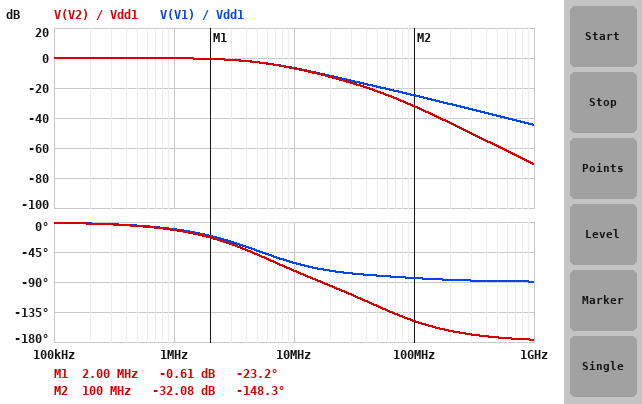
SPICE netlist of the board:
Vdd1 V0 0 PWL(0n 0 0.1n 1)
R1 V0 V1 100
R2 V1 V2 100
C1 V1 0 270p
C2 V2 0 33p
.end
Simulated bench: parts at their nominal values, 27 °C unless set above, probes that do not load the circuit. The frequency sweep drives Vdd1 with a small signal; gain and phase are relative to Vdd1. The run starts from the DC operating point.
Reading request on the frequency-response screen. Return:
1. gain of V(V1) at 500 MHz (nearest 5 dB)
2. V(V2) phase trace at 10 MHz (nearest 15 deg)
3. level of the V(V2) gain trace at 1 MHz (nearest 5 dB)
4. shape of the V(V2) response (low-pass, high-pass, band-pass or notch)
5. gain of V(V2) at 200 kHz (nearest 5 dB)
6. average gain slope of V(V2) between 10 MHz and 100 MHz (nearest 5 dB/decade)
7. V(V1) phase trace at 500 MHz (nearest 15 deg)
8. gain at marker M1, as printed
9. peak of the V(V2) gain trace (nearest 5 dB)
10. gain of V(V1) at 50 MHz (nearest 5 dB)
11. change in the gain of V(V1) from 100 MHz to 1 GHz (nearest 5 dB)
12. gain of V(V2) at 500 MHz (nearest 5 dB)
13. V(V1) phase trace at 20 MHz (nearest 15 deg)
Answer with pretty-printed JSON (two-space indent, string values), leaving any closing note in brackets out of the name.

{
  "gain of V(V1) at 500 MHz": "-40 dB",
  "V(V2) phase trace at 10 MHz": "-75 deg",
  "level of the V(V2) gain trace at 1 MHz": "0 dB",
  "shape of the V(V2) response": "low-pass",
  "gain of V(V2) at 200 kHz": "0 dB",
  "average gain slope of V(V2) between 10 MHz and 100 MHz": "-25 dB/decade",
  "V(V1) phase trace at 500 MHz": "-90 deg",
  "gain at marker M1, as printed": "-0.61 dB",
  "peak of the V(V2) gain trace": "0 dB",
  "gain of V(V1) at 50 MHz": "-20 dB",
  "change in the gain of V(V1) from 100 MHz to 1 GHz": "-20 dB",
  "gain of V(V2) at 500 MHz": "-60 dB",
  "V(V1) phase trace at 20 MHz": "-75 deg"
}
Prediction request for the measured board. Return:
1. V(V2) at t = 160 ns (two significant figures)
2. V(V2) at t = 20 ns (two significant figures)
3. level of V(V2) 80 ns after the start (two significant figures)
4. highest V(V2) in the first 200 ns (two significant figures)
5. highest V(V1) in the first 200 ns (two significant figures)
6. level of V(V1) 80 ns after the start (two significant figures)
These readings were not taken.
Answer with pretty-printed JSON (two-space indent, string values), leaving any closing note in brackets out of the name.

{
  "V(V2) at t = 160 ns": "990 mV",
  "V(V2) at t = 20 ns": "420 mV",
  "level of V(V2) 80 ns after the start": "920 mV",
  "highest V(V2) in the first 200 ns": "1.0 V",
  "highest V(V1) in the first 200 ns": "1.0 V",
  "level of V(V1) 80 ns after the start": "930 mV"
}
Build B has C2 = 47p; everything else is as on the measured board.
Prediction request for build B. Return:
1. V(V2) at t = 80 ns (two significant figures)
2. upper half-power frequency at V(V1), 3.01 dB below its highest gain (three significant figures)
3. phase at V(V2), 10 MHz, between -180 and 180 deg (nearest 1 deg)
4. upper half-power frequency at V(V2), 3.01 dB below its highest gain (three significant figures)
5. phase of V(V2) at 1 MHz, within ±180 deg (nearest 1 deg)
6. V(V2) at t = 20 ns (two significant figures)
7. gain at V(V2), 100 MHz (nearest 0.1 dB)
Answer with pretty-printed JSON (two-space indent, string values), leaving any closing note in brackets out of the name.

{
  "V(V2) at t = 80 ns": "900 mV",
  "upper half-power frequency at V(V1), 3.01 dB below its highest gain": "4.93 MHz",
  "phase at V(V2), 10 MHz, between -180 and 180 deg": "-78 deg",
  "upper half-power frequency at V(V2), 3.01 dB below its highest gain": "4.83 MHz",
  "phase of V(V2) at 1 MHz, within ±180 deg": "-13 deg",
  "V(V2) at t = 20 ns": "390 mV",
  "gain at V(V2), 100 MHz": "-34.7 dB"
}
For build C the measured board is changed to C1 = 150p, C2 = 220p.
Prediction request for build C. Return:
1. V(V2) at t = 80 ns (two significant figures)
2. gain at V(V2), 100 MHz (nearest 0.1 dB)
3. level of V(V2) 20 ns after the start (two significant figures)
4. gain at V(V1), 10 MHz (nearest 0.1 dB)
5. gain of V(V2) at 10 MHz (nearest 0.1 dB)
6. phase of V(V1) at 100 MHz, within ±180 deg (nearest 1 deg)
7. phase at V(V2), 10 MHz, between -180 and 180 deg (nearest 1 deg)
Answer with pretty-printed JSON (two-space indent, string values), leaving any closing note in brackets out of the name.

{
  "V(V2) at t = 80 ns": "750 mV",
  "gain at V(V2), 100 MHz": "-42.6 dB",
  "level of V(V2) 20 ns after the start": "230 mV",
  "gain at V(V1), 10 MHz": "-6.8 dB",
  "gain of V(V2) at 10 MHz": "-11.4 dB",
  "phase of V(V1) at 100 MHz, within ±180 deg": "-78 deg",
  "phase at V(V2), 10 MHz, between -180 and 180 deg": "-95 deg"
}
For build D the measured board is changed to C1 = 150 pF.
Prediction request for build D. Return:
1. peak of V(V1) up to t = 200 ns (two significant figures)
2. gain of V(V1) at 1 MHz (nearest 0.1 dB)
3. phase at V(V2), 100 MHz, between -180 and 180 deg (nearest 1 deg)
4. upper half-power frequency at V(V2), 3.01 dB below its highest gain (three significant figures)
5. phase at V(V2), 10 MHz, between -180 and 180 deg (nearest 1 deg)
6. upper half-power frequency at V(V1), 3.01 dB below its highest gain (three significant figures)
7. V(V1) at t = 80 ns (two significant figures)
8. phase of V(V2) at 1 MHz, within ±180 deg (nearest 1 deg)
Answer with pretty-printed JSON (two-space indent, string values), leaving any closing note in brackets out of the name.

{
  "peak of V(V1) up to t = 200 ns": "1.0 V",
  "gain of V(V1) at 1 MHz": "-0.1 dB",
  "phase at V(V2), 100 MHz, between -180 and 180 deg": "-144 deg",
  "upper half-power frequency at V(V2), 3.01 dB below its highest gain": "8.23 MHz",
  "phase at V(V2), 10 MHz, between -180 and 180 deg": "-59 deg",
  "upper half-power frequency at V(V1), 3.01 dB below its highest gain": "8.47 MHz",
  "V(V1) at t = 80 ns": "990 mV",
  "phase of V(V2) at 1 MHz, within ±180 deg": "-8 deg"
}
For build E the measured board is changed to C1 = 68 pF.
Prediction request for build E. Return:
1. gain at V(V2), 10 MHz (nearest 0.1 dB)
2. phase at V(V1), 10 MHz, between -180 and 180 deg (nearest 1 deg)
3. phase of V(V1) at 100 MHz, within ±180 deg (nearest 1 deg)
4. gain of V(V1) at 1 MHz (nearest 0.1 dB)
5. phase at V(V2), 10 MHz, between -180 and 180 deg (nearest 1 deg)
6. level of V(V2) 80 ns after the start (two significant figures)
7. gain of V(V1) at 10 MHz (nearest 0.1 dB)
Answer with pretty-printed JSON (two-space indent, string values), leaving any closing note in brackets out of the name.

{
  "gain at V(V2), 10 MHz": "-1.9 dB",
  "phase at V(V1), 10 MHz, between -180 and 180 deg": "-31 deg",
  "phase of V(V1) at 100 MHz, within ±180 deg": "-69 deg",
  "gain of V(V1) at 1 MHz": "0 dB",
  "phase at V(V2), 10 MHz, between -180 and 180 deg": "-43 deg",
  "level of V(V2) 80 ns after the start": "1.0 V",
  "gain of V(V1) at 10 MHz": "-1.7 dB"
}
